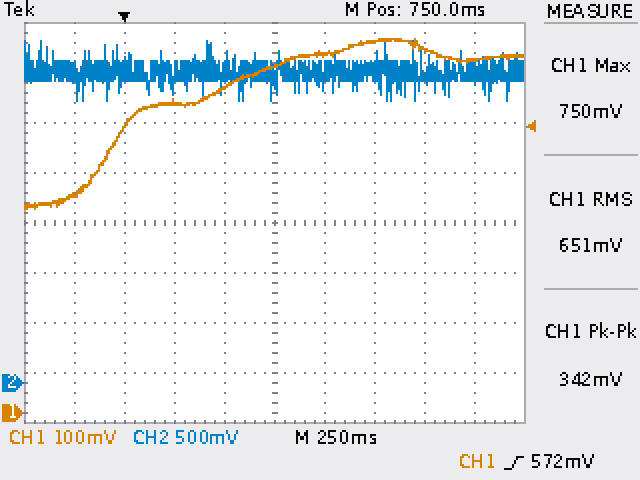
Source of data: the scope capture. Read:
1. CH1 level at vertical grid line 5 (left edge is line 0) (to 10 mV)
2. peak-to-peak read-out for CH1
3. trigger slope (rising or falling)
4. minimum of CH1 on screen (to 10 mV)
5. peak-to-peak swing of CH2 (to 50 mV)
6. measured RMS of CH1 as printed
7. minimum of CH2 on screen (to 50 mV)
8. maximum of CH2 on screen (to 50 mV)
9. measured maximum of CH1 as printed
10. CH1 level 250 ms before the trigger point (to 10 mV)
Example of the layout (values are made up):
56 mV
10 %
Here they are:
690 mV
342 mV
rising
410 mV
600 mV
651 mV
2.80 V
3.40 V
750 mV
440 mV
